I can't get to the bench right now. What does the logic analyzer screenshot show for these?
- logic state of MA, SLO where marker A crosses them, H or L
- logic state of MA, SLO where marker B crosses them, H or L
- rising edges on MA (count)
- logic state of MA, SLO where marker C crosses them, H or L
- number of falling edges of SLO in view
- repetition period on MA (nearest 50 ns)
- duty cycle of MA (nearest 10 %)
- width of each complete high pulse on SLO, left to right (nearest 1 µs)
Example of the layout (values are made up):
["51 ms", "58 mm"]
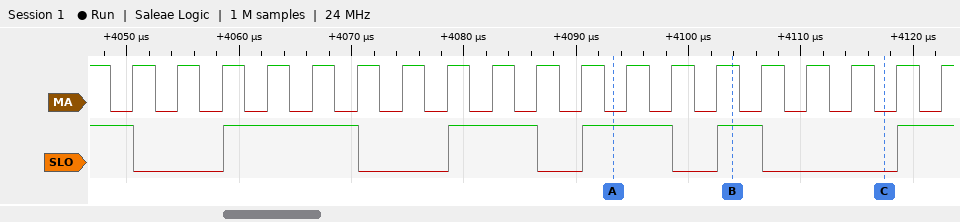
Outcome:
["MA=L, SLO=H", "MA=H, SLO=H", "19", "MA=L, SLO=L", "5", "4000 ns", "50 %", "12 µs, 8 µs, 8 µs, 4 µs"]
